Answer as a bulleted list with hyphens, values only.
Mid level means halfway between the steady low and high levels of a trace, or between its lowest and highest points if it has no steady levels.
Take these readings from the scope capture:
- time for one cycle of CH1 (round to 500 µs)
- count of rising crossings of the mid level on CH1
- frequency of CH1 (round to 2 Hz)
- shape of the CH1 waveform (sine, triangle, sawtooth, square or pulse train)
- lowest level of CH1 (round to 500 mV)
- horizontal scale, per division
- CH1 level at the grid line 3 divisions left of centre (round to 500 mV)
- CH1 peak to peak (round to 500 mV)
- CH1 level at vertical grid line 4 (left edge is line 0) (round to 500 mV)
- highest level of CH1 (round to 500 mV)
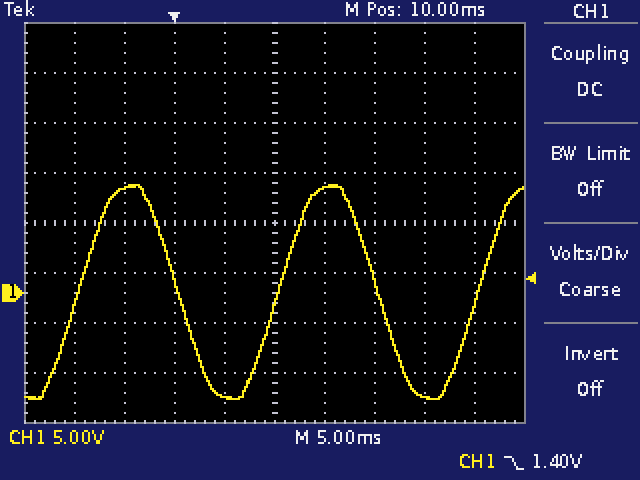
- 20.0 ms
- 3
- 50 Hz
- sine
- -10.5 V
- 5 ms
- 10.5 V
- 21.5 V
- -10.5 V
- 11.0 V
